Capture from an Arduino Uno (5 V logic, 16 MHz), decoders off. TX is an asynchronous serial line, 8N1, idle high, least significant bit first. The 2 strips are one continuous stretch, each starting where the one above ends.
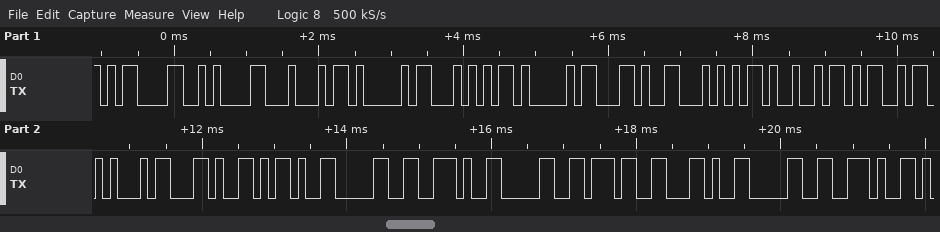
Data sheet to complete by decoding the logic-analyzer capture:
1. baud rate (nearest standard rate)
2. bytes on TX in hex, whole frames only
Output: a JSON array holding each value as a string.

["9600 baud", "0x0D 0x0A 0x44 0x41 0x54 0x41 0x2C 0x54 0x49 0x4D 0x45 0x2C 0x2D 0x30 0x2E 0x30 0x37 0x2C 0x30 0x2E"]
